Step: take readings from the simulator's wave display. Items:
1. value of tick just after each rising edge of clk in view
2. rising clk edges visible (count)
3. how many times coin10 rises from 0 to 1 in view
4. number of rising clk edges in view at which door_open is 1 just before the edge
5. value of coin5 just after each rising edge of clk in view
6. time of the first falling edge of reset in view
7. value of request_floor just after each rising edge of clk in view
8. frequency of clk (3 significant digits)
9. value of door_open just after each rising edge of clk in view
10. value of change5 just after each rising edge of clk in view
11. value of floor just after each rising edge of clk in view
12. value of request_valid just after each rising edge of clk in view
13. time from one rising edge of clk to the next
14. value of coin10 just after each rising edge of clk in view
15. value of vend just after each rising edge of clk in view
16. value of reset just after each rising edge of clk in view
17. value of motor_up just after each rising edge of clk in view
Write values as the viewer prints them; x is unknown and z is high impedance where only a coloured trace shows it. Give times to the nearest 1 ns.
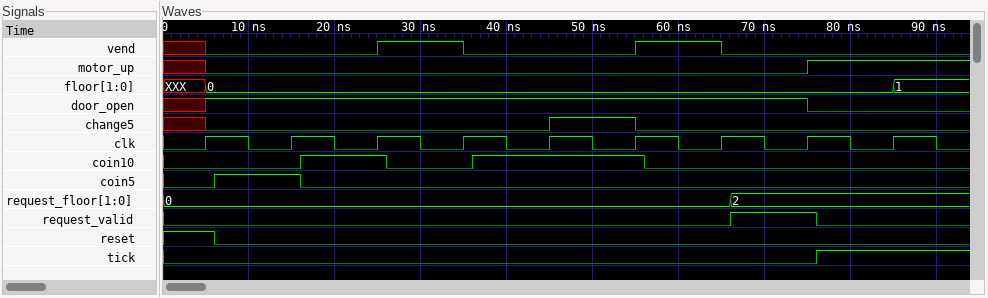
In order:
0 0 0 0 0 0 0 0 1
9
2
7
0 1 0 0 0 0 0 0 0
6 ns
0, 0, 0, 0, 0, 0, 0, 2, 2
100 MHz
1 1 1 1 1 1 1 0 0
0 0 0 0 1 0 0 0 0
0, 0, 0, 0, 0, 0, 0, 0, 1
0 0 0 0 0 0 0 1 0
10 ns
0 0 1 0 1 1 0 0 0
0 0 1 0 0 1 0 0 0
1 0 0 0 0 0 0 0 0
0 0 0 0 0 0 0 1 1
